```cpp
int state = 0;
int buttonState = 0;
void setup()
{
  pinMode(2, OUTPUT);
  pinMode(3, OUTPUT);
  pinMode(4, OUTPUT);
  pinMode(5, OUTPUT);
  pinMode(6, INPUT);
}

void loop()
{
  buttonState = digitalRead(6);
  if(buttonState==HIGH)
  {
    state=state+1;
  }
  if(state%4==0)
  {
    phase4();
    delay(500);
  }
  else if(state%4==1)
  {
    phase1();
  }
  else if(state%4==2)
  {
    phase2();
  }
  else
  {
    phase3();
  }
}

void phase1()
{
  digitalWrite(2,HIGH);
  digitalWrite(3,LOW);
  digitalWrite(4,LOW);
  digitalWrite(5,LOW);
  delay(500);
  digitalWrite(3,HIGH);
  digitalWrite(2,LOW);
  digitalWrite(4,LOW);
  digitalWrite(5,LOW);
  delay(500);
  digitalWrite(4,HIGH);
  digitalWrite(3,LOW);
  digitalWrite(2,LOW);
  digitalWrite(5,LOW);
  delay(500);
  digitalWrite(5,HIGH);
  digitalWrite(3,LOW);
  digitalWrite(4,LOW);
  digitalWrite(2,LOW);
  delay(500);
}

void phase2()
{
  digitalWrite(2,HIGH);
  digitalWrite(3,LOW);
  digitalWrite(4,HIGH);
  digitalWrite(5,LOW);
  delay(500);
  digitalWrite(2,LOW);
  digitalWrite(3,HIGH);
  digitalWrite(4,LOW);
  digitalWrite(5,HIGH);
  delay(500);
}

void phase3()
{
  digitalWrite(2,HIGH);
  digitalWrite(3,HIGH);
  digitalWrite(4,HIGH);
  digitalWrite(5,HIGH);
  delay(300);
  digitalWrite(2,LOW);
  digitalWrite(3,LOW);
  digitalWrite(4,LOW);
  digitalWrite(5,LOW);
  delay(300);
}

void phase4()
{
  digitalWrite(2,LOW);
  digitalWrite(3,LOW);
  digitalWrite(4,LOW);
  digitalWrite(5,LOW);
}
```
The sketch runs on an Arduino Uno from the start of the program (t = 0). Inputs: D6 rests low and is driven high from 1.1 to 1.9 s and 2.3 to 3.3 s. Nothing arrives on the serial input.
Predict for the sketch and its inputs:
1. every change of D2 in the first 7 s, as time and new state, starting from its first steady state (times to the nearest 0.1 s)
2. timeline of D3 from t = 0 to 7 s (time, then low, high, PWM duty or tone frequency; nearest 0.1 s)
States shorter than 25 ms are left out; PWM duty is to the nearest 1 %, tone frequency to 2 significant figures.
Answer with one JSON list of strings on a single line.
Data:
["0 s low; 1.5 s high; 2 s low; 3.5 s high; 4 s low; 5.5 s high; 6 s low", "0 s low; 2 s high; 2.5 s low; 4 s high; 4.5 s low; 6 s high; 6.5 s low"]
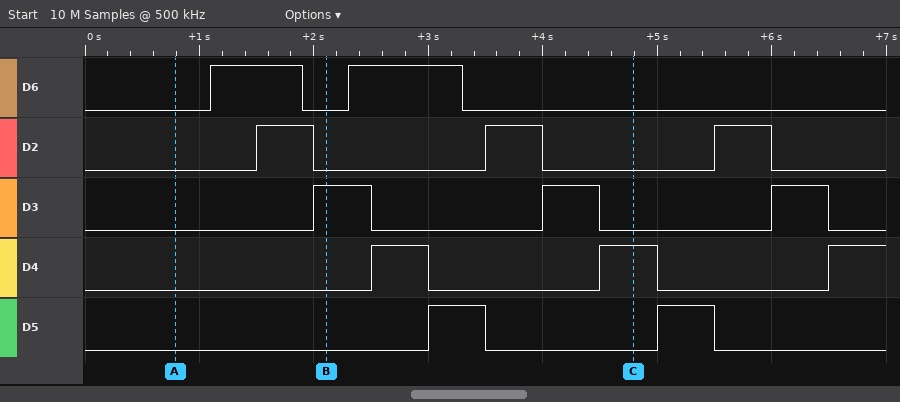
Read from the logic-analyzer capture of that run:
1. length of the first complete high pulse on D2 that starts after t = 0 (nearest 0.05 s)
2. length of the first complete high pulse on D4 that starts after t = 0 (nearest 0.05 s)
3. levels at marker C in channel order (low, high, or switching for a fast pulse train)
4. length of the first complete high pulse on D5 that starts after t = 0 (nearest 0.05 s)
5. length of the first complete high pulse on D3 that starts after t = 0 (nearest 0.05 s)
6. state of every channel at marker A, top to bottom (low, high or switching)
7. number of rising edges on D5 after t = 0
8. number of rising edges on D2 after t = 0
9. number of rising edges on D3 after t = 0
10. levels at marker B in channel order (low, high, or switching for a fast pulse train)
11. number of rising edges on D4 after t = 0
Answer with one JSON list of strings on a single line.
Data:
["0.50 s", "0.50 s", "D6 low, D2 low, D3 low, D4 high, D5 low", "0.50 s", "0.50 s", "D6 low, D2 low, D3 low, D4 low, D5 low", "2", "3", "3", "D6 low, D2 low, D3 high, D4 low, D5 low", "3"]
